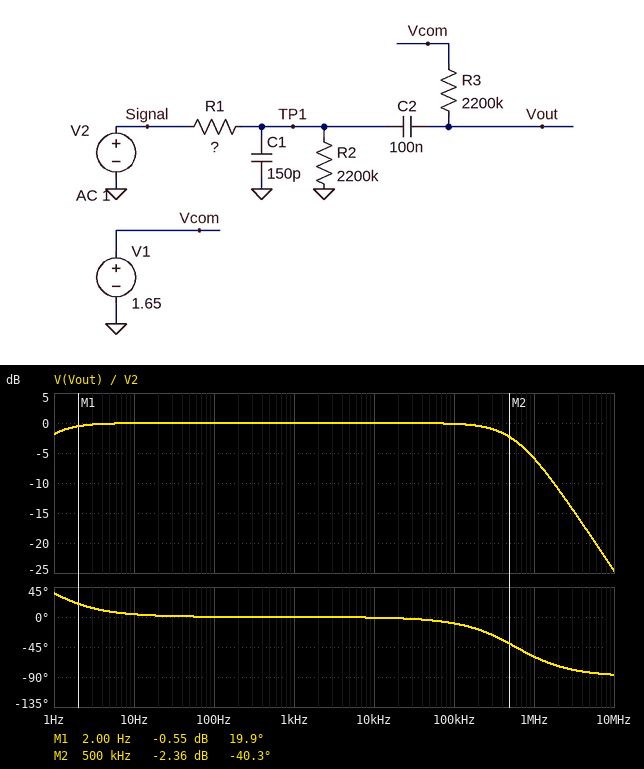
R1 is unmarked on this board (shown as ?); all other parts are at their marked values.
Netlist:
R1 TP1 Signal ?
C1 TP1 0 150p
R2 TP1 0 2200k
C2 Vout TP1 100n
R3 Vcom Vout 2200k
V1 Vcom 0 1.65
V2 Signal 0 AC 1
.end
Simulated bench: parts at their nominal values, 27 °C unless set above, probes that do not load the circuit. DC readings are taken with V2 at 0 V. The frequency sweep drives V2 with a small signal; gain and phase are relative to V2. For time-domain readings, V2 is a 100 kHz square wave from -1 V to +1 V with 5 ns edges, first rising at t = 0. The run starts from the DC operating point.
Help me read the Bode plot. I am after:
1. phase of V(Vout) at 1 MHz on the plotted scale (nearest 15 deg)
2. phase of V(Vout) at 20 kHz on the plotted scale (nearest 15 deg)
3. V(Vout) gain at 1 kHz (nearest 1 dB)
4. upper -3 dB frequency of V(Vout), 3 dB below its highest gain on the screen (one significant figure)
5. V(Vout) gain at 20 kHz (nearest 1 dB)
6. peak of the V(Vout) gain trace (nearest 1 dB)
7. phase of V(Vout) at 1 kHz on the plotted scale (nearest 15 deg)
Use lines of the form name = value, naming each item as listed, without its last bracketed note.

phase of V(Vout) at 1 MHz on the plotted scale = -60 deg
phase of V(Vout) at 20 kHz on the plotted scale = 0 deg
V(Vout) gain at 1 kHz = 0 dB
upper -3 dB frequency of V(Vout), 3 dB below its highest gain on the screen = 600 kHz
V(Vout) gain at 20 kHz = 0 dB
peak of the V(Vout) gain trace = 0 dB
phase of V(Vout) at 1 kHz on the plotted scale = 0 deg
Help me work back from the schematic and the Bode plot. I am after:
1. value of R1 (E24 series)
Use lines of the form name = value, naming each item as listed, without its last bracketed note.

value of R1 = 1.8 kΩ
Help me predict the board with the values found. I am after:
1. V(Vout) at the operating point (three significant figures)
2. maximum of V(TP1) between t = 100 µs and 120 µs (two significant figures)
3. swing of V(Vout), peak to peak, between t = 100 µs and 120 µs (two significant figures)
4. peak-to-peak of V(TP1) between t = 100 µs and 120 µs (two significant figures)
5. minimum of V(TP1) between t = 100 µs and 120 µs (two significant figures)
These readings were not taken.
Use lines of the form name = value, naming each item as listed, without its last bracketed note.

V(Vout) at the operating point = 1.65 V
maximum of V(TP1) between t = 100 µs and 120 µs = 1.0 V
swing of V(Vout), peak to peak, between t = 100 µs and 120 µs = 2.0 V
peak-to-peak of V(TP1) between t = 100 µs and 120 µs = 2.0 V
minimum of V(TP1) between t = 100 µs and 120 µs = -1.0 V
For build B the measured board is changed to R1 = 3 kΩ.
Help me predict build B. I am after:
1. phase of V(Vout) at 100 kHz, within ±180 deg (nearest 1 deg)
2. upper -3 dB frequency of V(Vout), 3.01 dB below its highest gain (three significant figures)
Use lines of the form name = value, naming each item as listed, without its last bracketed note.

phase of V(Vout) at 100 kHz, within ±180 deg = -16 deg
upper -3 dB frequency of V(Vout), 3.01 dB below its highest gain = 355 kHz
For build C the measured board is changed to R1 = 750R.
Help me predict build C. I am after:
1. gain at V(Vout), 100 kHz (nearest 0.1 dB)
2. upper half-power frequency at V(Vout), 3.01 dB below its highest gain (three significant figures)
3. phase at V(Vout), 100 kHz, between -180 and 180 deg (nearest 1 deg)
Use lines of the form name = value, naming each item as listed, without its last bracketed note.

gain at V(Vout), 100 kHz = 0 dB
upper half-power frequency at V(Vout), 3.01 dB below its highest gain = 1.42 MHz
phase at V(Vout), 100 kHz, between -180 and 180 deg = -4 deg
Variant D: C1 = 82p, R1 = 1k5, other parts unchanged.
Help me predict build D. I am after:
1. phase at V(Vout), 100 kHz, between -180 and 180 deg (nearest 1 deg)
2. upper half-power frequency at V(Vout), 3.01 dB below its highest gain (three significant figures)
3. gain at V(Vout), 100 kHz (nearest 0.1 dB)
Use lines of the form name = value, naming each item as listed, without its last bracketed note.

phase at V(Vout), 100 kHz, between -180 and 180 deg = -4 deg
upper half-power frequency at V(Vout), 3.01 dB below its highest gain = 1.30 MHz
gain at V(Vout), 100 kHz = 0 dB
